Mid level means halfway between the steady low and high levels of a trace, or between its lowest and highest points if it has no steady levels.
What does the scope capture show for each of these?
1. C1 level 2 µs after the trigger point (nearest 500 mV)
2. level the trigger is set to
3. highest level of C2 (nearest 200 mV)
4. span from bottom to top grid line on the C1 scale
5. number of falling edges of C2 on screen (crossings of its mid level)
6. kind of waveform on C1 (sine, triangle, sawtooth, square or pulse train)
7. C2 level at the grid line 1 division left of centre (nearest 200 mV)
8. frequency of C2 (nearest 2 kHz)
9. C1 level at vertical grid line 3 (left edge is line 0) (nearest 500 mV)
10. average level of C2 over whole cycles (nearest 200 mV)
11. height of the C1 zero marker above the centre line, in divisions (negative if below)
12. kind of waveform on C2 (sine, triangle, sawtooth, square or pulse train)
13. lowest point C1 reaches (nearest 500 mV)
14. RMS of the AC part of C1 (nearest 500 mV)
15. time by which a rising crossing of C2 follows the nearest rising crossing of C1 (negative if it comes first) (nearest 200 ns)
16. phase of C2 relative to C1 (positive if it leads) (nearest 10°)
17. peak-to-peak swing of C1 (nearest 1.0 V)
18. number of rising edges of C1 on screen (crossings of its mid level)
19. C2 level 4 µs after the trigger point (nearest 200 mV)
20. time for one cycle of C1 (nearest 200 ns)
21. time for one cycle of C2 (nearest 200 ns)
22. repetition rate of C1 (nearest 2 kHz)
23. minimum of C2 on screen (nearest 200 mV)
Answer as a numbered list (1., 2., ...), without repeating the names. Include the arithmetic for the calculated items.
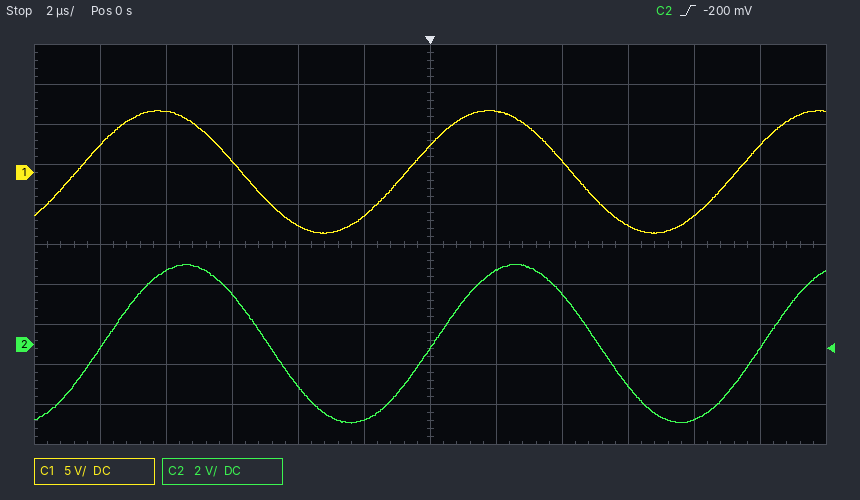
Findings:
1. 7.5 V
2. -200 mV
3. 4.0 V
4. 50 V
5. 2
6. sine
7. -3.8 V
8. 1 / 10.0 µs ≈ 100 kHz
9. 1.5 V
10. (4.0 V + (-4.0 V)) / 2 ≈ 0.0 V
11. +1.8 div
12. sine
13. -7.5 V
14. 15.0 V / (2√2) ≈ 5.30 V, so 5.5 V to the nearest 500 mV
15. +800 ns
16. −360° × (+800 ns) / 10.0 µs ≈ -28.8°, so -30° to the nearest 10°
17. 15.0 V
18. 3
19. 2.6 V
20. 10.0 µs
21. 10.0 µs
22. 1 / 10.0 µs ≈ 100 kHz
23. -4.0 V
